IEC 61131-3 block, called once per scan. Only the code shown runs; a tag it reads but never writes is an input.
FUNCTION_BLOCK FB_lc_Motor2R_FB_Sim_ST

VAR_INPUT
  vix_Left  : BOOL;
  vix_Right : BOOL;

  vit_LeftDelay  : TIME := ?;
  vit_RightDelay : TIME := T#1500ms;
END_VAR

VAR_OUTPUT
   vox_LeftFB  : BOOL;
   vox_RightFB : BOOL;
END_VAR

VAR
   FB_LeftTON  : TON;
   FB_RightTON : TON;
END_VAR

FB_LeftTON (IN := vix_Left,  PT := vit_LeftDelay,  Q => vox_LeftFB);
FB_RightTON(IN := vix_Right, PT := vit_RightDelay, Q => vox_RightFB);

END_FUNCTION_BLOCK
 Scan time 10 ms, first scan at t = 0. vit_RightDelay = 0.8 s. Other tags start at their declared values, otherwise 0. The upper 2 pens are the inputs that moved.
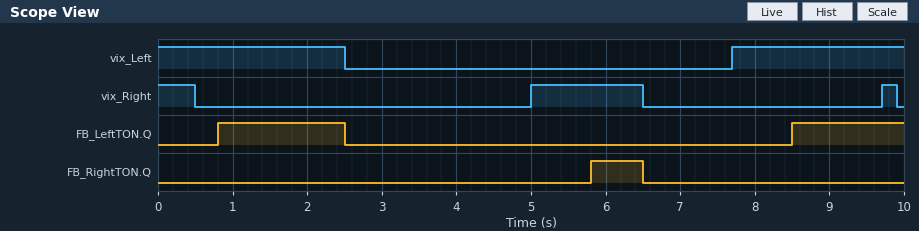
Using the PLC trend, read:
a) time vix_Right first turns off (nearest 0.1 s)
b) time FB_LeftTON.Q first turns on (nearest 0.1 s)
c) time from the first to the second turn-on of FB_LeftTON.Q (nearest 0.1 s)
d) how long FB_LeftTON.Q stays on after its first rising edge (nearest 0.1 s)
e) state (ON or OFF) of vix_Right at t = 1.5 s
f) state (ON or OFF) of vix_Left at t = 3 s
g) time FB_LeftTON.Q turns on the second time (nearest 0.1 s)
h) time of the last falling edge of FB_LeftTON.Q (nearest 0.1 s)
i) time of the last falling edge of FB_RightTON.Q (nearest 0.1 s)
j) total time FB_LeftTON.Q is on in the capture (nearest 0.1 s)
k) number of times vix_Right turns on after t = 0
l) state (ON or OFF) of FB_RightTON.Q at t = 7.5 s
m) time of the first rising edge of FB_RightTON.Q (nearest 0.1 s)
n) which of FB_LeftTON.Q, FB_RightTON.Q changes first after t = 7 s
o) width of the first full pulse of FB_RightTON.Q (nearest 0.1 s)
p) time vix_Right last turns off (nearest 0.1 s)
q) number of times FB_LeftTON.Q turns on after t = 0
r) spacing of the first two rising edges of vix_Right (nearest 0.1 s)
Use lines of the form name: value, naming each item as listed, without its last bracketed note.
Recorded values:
time vix_Right first turns off: 0.5 s
time FB_LeftTON.Q first turns on: 0.8 s
time from the first to the second turn-on of FB_LeftTON.Q: 7.7 s
how long FB_LeftTON.Q stays on after its first rising edge: 1.7 s
state (ON or OFF) of vix_Right at t = 1.5 s: OFF
state (ON or OFF) of vix_Left at t = 3 s: OFF
time FB_LeftTON.Q turns on the second time: 8.5 s
time of the last falling edge of FB_LeftTON.Q: 2.5 s
time of the last falling edge of FB_RightTON.Q: 6.5 s
total time FB_LeftTON.Q is on in the capture: 3.2 s
number of times vix_Right turns on after t = 0: 2
state (ON or OFF) of FB_RightTON.Q at t = 7.5 s: OFF
time of the first rising edge of FB_RightTON.Q: 5.8 s
which of FB_LeftTON.Q, FB_RightTON.Q changes first after t = 7 s: FB_LeftTON.Q
width of the first full pulse of FB_RightTON.Q: 0.7 s
time vix_Right last turns off: 9.9 s
number of times FB_LeftTON.Q turns on after t = 0: 2
spacing of the first two rising edges of vix_Right: 4.7 s
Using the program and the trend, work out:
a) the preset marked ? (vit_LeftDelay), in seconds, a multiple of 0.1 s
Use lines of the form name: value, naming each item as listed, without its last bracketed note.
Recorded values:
the preset marked ? (vit_LeftDelay), in seconds, a multiple of 0.1 s: 0.8 s
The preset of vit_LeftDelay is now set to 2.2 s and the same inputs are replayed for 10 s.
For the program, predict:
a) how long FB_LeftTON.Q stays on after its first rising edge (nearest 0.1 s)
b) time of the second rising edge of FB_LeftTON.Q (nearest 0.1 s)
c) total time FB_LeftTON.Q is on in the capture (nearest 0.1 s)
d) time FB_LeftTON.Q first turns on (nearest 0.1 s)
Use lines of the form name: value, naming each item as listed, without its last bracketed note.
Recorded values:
how long FB_LeftTON.Q stays on after its first rising edge: 0.3 s
time of the second rising edge of FB_LeftTON.Q: 9.9 s
total time FB_LeftTON.Q is on in the capture: 0.4 s
time FB_LeftTON.Q first turns on: 2.2 s
